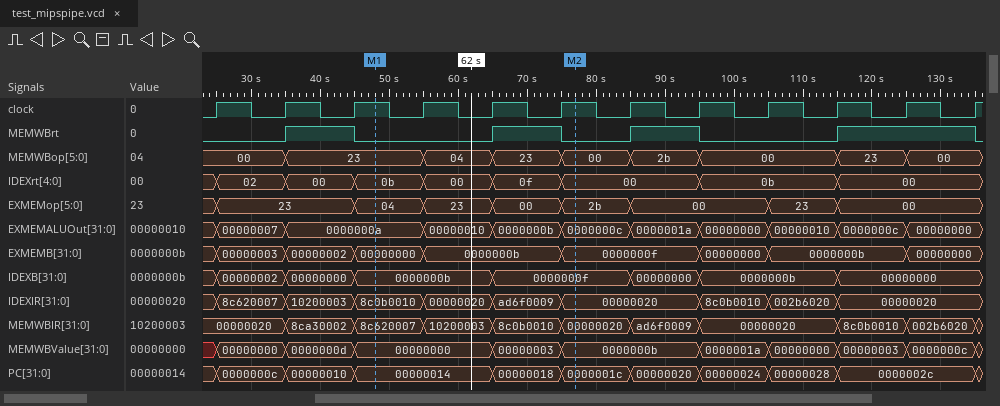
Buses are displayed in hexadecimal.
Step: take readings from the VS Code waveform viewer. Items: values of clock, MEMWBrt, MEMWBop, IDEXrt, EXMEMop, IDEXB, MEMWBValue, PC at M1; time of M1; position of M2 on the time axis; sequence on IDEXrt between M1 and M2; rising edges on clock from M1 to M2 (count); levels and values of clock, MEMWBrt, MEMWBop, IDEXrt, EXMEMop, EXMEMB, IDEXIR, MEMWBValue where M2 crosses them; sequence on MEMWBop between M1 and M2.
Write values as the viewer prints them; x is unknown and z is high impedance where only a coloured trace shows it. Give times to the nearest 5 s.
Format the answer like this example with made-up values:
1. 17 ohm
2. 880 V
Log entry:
1. clock=1, MEMWBrt=0, MEMWBop=23, IDEXrt=0b, EXMEMop=04, IDEXB=0000000b, MEMWBValue=00000000, PC=00000014
2. 50 s
3. 75 s
4. 0b, 00, 0f, 00
5. 3
6. clock=1, MEMWBrt=0, MEMWBop=00, IDEXrt=00, EXMEMop=2b, EXMEMB=0000000f, IDEXIR=00000020, MEMWBValue=0000000b
7. 23, 04, 23, 00
